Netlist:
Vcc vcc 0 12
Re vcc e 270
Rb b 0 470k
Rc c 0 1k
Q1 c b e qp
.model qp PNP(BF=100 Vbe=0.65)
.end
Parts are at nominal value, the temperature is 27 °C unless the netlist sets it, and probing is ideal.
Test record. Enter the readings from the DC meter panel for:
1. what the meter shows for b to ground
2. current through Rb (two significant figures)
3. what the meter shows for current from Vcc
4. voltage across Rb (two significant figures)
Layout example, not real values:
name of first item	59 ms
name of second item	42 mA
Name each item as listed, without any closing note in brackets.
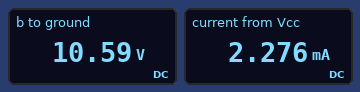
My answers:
what the meter shows for b to ground	10.59 V
current through Rb	23 µA
what the meter shows for current from Vcc	2.276 mA
voltage across Rb	11 V
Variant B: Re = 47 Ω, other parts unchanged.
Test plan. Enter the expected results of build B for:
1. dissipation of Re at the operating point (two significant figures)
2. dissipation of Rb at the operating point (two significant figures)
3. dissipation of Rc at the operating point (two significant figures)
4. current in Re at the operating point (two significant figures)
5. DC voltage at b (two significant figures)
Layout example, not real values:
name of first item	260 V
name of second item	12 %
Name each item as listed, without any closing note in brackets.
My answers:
dissipation of Re at the operating point	270 µW
dissipation of Rb at the operating point	260 µW
dissipation of Rc at the operating point	5.6 mW
current in Re at the operating point	2.4 mA
DC voltage at b	11 V
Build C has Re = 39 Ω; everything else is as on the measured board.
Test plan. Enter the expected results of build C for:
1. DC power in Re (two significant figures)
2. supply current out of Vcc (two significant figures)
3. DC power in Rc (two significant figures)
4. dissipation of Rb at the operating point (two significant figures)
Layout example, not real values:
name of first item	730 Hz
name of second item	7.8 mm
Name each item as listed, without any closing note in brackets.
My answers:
DC power in Re	220 µW
supply current out of Vcc	2.4 mA
DC power in Rc	5.6 mW
dissipation of Rb at the operating point	260 µW
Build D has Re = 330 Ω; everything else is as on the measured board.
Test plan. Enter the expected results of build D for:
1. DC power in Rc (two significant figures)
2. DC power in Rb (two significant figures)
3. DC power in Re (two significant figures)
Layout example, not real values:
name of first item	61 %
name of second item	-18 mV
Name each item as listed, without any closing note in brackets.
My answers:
DC power in Rc	5.0 mW
DC power in Rb	230 µW
DC power in Re	1.7 mW
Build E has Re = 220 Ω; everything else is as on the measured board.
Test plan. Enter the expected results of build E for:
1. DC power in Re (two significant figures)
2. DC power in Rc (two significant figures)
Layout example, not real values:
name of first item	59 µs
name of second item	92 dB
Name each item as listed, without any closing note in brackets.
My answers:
DC power in Re	1.2 mW
DC power in Rc	5.2 mW
